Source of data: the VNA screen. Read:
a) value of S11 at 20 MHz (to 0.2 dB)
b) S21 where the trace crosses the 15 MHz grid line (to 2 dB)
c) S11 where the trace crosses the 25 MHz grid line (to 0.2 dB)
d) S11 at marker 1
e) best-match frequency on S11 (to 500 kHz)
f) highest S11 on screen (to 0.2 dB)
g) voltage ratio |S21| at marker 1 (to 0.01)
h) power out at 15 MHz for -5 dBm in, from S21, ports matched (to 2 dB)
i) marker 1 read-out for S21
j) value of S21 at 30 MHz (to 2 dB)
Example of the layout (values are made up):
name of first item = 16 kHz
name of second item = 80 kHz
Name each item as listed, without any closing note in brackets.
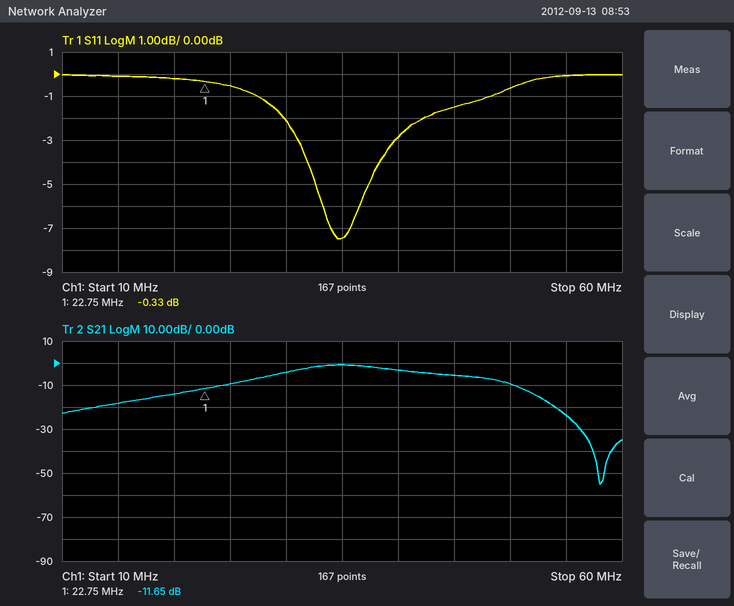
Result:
value of S11 at 20 MHz = -0.2 dB
S21 where the trace crosses the 15 MHz grid line = -18 dB
S11 where the trace crosses the 25 MHz grid line = -0.6 dB
S11 at marker 1 = -0.33 dB
best-match frequency on S11 = 34.5 MHz
highest S11 on screen = 0.0 dB
voltage ratio |S21| at marker 1 = 0.26
power out at 15 MHz for -5 dBm in, from S21, ports matched = -24 dBm
marker 1 read-out for S21 = -11.65 dB
value of S21 at 30 MHz = -4 dB
